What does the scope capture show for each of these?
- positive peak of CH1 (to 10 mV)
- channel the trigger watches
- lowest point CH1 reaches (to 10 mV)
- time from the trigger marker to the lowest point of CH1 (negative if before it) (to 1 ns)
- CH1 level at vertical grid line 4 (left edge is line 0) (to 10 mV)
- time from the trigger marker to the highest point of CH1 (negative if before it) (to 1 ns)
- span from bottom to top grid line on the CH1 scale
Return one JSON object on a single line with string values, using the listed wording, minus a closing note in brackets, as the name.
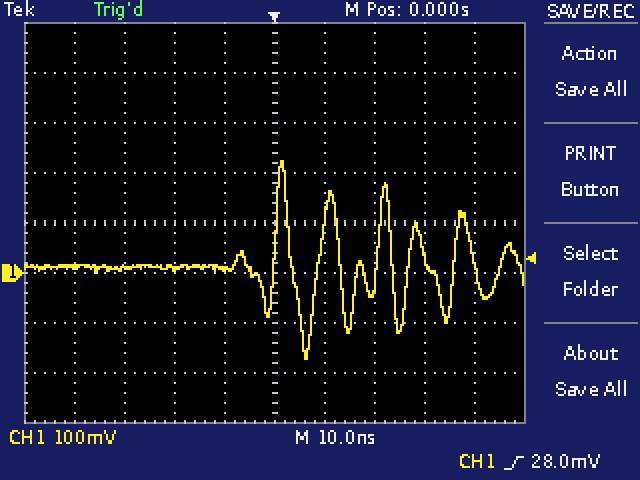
{"positive peak of CH1": "220 mV", "channel the trigger watches": "CH1", "lowest point CH1 reaches": "-170 mV", "time from the trigger marker to the lowest point of CH1 (negative if before it)": "+6 ns", "CH1 level at vertical grid line 4 (left edge is line 0)": "10 mV", "time from the trigger marker to the highest point of CH1 (negative if before it)": "+2 ns", "span from bottom to top grid line on the CH1 scale": "800 mV"}
